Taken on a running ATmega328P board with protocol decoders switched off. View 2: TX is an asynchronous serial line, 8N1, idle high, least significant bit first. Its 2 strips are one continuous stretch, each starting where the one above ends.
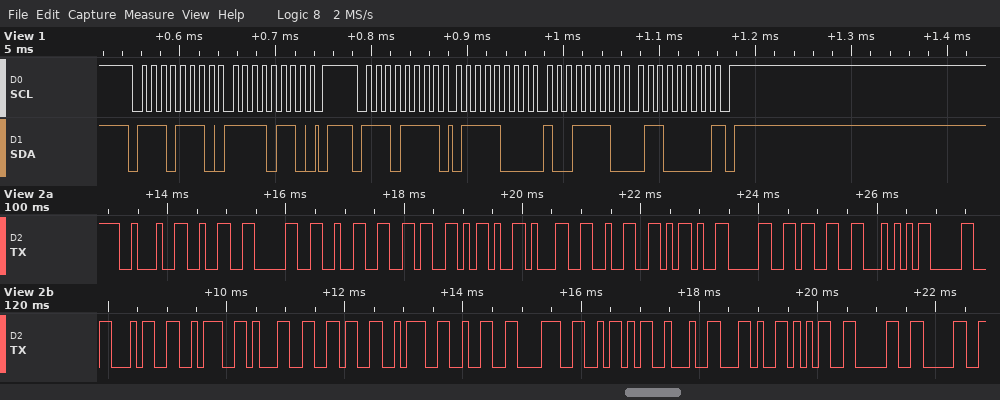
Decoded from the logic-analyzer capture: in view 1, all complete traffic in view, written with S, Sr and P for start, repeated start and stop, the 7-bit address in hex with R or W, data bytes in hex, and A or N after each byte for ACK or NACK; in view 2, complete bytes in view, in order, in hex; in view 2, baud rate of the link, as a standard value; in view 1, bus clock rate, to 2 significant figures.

S 77W A F6 A P S 77R A 78 A 9E A 60 N P
0x22 0x32 0x30 0x32 0x36 0x2D 0x31 0x32 0x2D 0x30 0x33 0x54 0x30 0x34 0x3A 0x31 0x36 0x3A 0x32 0x38 0x5A 0x22 0x2C 0x35 0x30 0x30
9600 baud
100 kHz
